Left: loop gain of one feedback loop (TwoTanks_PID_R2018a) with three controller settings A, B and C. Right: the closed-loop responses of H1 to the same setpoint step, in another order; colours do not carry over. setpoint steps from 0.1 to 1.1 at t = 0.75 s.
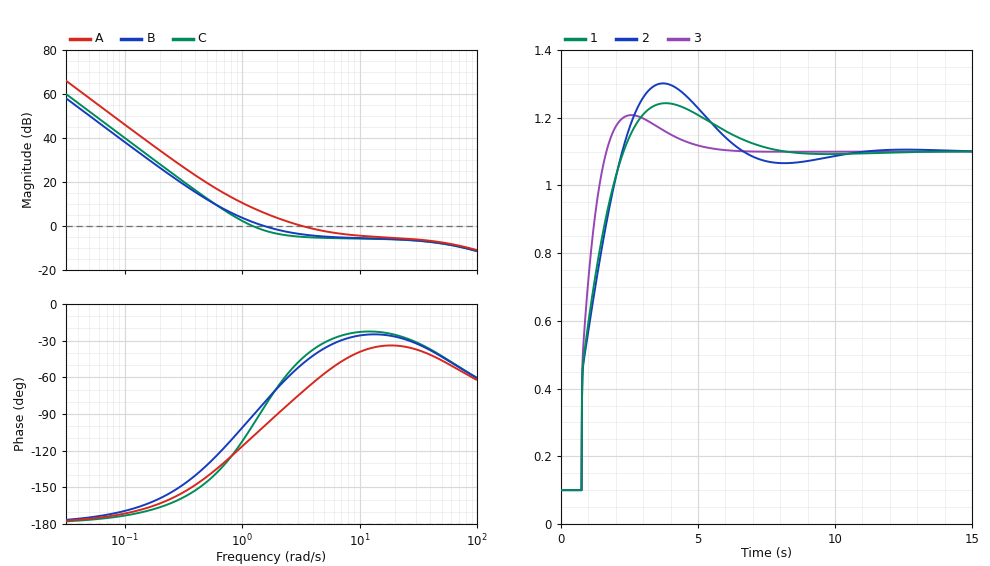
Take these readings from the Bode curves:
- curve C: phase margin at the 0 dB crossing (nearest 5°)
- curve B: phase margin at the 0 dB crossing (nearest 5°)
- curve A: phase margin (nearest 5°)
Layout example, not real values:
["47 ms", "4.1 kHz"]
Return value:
["80°", "100°", "110°"]
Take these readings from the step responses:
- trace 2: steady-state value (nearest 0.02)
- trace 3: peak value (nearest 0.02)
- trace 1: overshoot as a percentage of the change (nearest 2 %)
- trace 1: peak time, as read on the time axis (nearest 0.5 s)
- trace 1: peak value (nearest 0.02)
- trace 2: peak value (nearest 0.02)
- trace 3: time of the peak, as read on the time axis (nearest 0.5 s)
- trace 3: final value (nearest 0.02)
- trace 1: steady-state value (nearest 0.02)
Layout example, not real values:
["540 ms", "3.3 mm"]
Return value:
["1.10", "1.20", "14 %", "4.0 s", "1.24", "1.30", "2.5 s", "1.10", "1.10"]
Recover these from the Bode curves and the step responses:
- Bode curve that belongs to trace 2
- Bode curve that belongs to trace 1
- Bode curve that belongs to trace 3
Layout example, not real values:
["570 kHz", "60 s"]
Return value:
["C", "B", "A"]
